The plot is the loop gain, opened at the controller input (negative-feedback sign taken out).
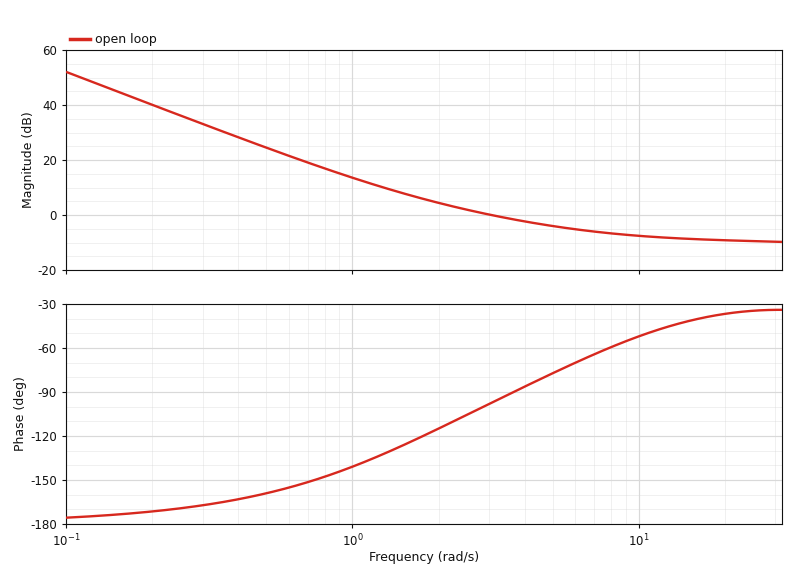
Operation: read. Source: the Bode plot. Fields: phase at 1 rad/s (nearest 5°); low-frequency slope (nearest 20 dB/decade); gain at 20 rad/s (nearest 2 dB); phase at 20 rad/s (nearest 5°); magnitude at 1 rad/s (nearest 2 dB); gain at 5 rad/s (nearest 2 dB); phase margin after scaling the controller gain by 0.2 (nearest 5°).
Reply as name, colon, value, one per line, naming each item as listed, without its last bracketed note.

phase at 1 rad/s: -140°
low-frequency slope: -40 dB/decade
gain at 20 rad/s: -10 dB
phase at 20 rad/s: -35°
magnitude at 1 rad/s: 14 dB
gain at 5 rad/s: -4 dB
phase margin after scaling the controller gain by 0.2: 40°
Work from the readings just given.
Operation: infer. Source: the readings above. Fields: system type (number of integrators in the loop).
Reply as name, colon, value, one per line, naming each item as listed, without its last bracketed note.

system type: 2
